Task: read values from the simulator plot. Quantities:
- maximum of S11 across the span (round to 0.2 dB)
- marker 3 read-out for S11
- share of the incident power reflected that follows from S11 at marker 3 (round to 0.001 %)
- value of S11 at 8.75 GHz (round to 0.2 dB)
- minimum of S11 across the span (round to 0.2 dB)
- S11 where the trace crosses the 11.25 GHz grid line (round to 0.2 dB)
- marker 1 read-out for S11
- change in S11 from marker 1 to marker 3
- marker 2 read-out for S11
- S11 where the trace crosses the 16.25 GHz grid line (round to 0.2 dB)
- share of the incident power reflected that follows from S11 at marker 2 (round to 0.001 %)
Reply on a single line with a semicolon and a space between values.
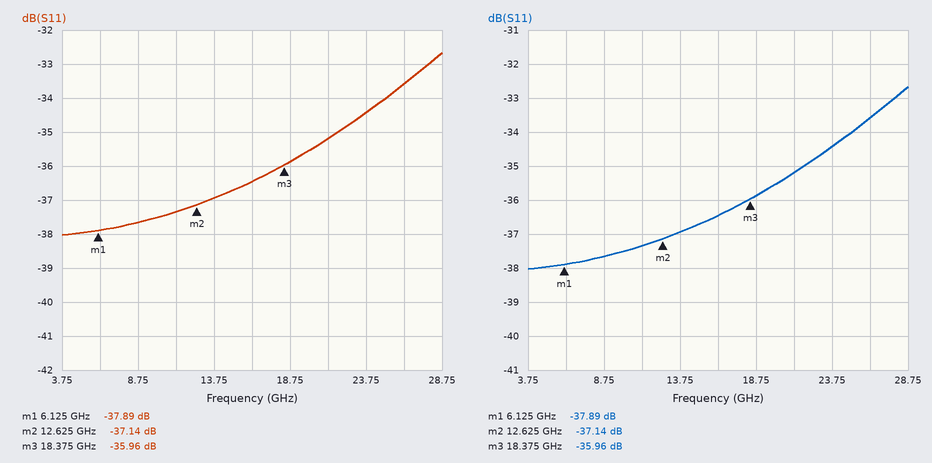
-32.6 dB; -35.96 dB; 0.025 %; -37.6 dB; -38.0 dB; -37.4 dB; -37.89 dB; 1.93 dB; -37.14 dB; -36.4 dB; 0.019 %
